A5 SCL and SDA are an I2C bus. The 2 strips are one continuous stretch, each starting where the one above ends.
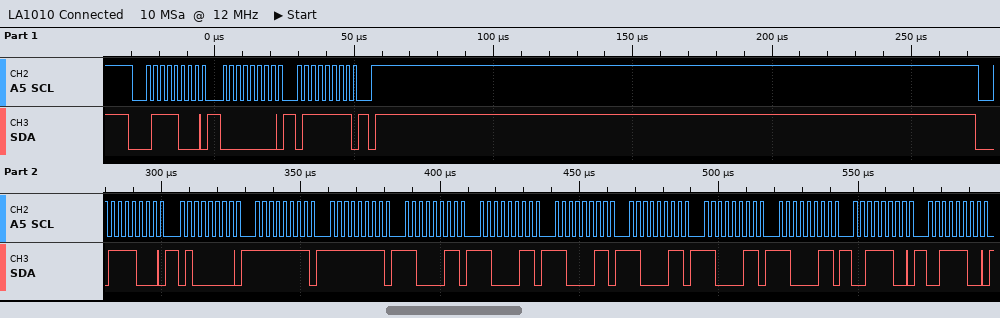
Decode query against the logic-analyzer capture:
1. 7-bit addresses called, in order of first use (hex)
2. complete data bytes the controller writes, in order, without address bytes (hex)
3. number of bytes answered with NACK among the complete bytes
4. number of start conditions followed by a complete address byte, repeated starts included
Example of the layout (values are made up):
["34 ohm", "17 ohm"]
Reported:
["0x3C", "00 7F 40 FF FF C3 C3 C3 C3 C3 C3 3C 3C", "0", "2"]
